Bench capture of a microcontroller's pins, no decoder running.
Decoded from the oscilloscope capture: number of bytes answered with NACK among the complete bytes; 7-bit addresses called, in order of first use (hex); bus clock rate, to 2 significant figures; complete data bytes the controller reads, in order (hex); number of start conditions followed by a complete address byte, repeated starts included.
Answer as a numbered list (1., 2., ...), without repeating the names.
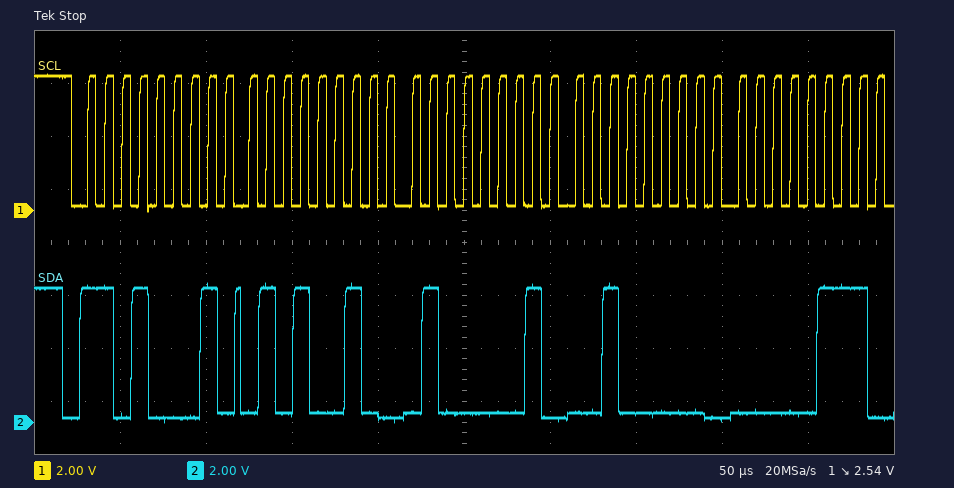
1. 0
2. 0x68
3. 100 kHz
4. 52 41 20 07
5. 1
